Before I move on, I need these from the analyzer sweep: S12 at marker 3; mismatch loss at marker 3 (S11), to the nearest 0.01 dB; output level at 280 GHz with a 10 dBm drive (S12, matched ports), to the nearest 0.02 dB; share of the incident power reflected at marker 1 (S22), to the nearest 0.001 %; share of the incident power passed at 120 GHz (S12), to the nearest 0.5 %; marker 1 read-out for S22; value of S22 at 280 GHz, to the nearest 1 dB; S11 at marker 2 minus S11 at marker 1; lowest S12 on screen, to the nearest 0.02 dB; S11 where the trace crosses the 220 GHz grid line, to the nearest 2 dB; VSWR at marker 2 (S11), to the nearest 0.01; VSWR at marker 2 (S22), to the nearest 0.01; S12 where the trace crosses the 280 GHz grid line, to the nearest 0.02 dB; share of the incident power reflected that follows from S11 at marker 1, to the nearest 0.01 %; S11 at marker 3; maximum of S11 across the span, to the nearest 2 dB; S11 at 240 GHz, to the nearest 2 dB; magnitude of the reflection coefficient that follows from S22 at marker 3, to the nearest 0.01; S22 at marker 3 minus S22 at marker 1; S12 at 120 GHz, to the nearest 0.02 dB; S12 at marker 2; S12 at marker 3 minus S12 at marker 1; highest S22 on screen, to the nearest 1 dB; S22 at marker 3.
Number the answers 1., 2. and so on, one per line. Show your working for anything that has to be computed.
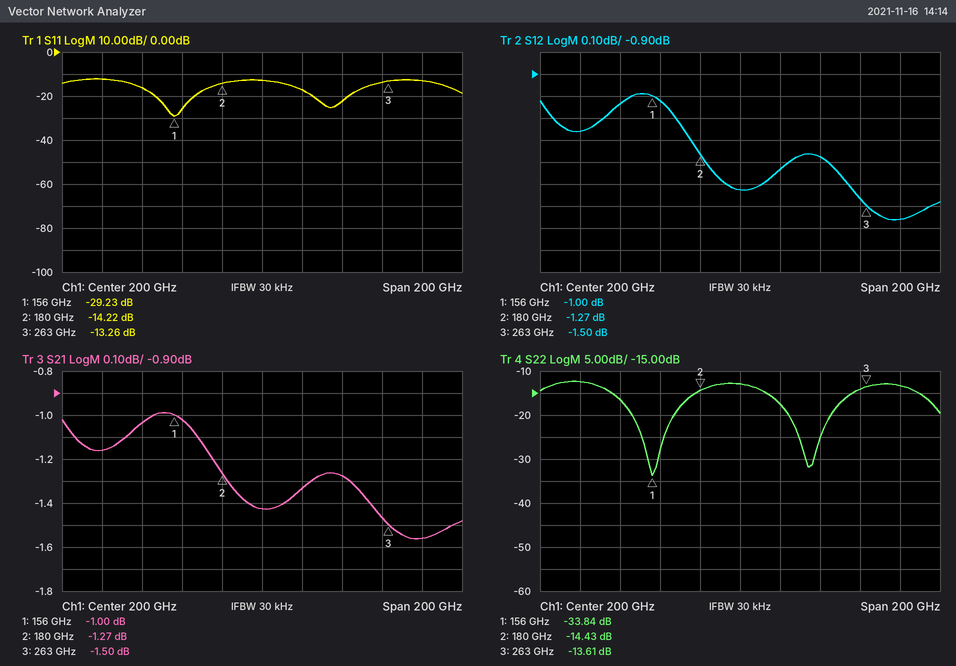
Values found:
1. -1.50 dB
2. −10 log10(1 − 10^(-13.26/10)) ≈ 0.21 dB
3. 10 dBm + (-1.56 dB) = 8.44 dBm
4. 10^(-33.84/10) ≈ 0.041 %
5. 10^(-1.16/10) ≈ 76.6 %, so 76.5 % to the nearest 0.5 %
6. -33.84 dB
7. -13 dB
8. -14.22 − (-29.23) = 15.01 dB
9. -1.56 dB
10. -18 dB
11. (1 + 0.1945)/(1 − 0.1945) ≈ 1.48
12. (1 + 0.1899)/(1 − 0.1899) ≈ 1.47
13. -1.56 dB
14. 10^(-29.23/10) ≈ 0.12 %
15. -13.26 dB
16. -12 dB
17. -22 dB
18. 10^(-13.61/20) ≈ 0.21
19. -13.61 − (-33.84) = 20.23 dB
20. -1.16 dB
21. -1.27 dB
22. -1.5 − (-1) = -0.50 dB
23. -12 dB
24. -13.61 dB
